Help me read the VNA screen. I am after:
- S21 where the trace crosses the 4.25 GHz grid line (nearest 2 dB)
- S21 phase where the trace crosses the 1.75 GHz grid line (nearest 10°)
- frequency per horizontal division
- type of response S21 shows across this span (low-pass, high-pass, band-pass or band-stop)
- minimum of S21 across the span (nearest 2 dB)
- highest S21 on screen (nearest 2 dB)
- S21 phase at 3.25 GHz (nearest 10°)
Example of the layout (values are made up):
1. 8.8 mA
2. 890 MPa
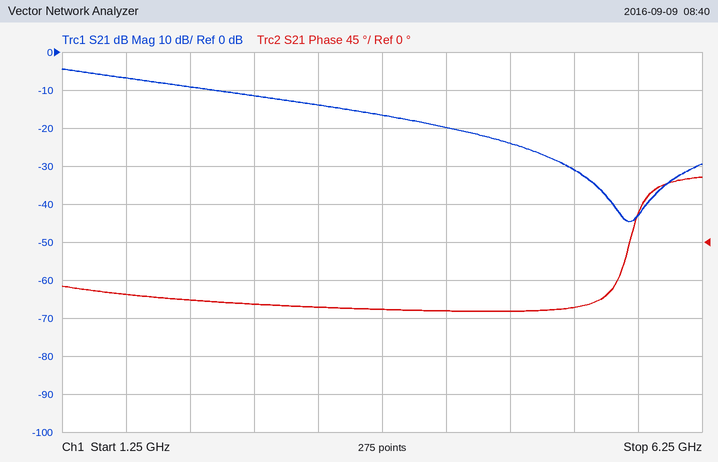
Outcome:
1. -20 dB
2. -60°
3. 500 MHz
4. low-pass
5. -44 dB
6. -4 dB
7. -80°
